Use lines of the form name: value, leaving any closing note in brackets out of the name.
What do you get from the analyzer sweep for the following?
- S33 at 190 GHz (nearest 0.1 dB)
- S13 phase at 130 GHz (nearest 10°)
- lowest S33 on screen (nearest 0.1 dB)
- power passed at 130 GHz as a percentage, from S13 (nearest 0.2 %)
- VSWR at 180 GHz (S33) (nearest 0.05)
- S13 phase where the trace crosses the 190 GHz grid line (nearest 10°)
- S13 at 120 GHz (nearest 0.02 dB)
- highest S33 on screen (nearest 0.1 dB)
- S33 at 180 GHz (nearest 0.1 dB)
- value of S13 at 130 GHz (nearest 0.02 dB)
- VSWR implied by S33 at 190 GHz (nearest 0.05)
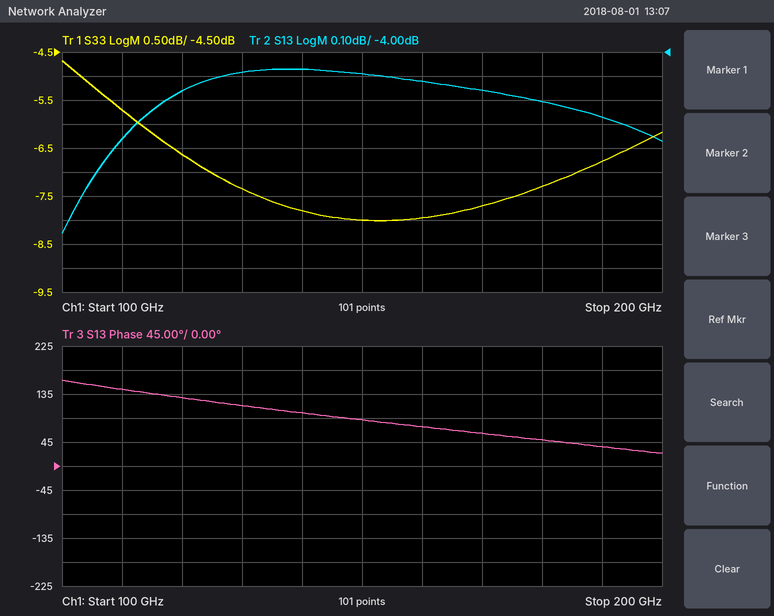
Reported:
S33 at 190 GHz: -6.8 dB
S13 phase at 130 GHz: 110°
lowest S33 on screen: -8.0 dB
power passed at 130 GHz as a percentage, from S13: 39.0 %
VSWR at 180 GHz (S33): 2.50
S13 phase where the trace crosses the 190 GHz grid line: 40°
S13 at 120 GHz: -4.16 dB
highest S33 on screen: -4.7 dB
S33 at 180 GHz: -7.3 dB
value of S13 at 130 GHz: -4.08 dB
VSWR implied by S33 at 190 GHz: 2.70
